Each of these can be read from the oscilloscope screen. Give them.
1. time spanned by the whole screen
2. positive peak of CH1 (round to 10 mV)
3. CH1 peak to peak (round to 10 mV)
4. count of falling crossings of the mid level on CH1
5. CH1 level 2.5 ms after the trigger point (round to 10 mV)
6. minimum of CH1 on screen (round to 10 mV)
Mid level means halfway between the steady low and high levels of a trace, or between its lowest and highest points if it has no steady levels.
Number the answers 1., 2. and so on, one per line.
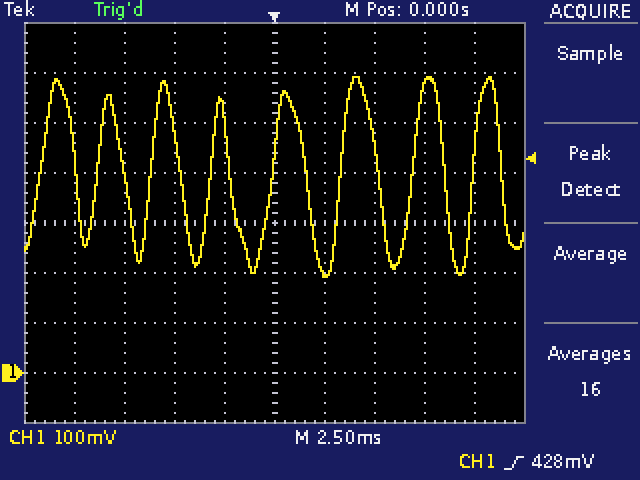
1. 25 ms
2. 590 mV
3. 400 mV
4. 8
5. 200 mV
6. 190 mV
